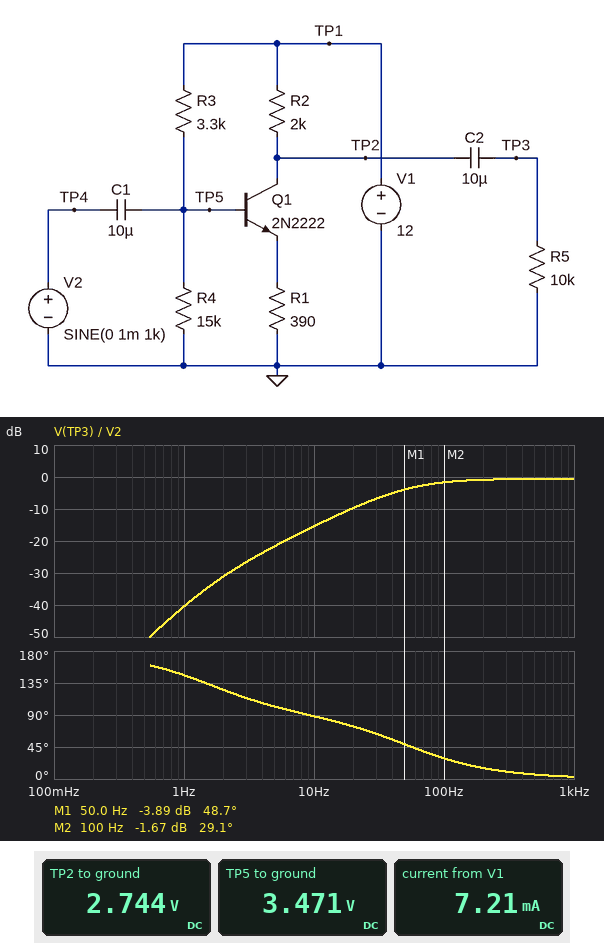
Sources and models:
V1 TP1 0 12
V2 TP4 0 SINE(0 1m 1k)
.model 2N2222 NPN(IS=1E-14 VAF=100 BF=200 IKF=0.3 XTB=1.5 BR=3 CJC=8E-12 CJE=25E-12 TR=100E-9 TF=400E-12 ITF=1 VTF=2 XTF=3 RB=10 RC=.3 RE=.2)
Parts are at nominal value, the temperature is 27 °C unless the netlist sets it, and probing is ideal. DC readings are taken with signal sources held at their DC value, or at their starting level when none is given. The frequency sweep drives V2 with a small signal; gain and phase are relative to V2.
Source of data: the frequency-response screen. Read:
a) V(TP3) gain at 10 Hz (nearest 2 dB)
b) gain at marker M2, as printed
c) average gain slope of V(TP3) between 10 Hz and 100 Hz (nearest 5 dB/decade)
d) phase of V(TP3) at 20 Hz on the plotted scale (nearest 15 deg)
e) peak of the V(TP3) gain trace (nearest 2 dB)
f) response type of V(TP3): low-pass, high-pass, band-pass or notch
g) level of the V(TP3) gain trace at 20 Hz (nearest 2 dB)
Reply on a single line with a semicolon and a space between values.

-16 dB; -1.67 dB; 15 dB/decade; 75 deg; 0 dB; high-pass; -10 dB
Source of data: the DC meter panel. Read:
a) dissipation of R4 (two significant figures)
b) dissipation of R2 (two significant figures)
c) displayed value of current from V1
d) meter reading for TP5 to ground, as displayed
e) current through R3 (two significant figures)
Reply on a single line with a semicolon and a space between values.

800 µW; 43 mW; 7.21 mA; 3.471 V; 2.6 mA
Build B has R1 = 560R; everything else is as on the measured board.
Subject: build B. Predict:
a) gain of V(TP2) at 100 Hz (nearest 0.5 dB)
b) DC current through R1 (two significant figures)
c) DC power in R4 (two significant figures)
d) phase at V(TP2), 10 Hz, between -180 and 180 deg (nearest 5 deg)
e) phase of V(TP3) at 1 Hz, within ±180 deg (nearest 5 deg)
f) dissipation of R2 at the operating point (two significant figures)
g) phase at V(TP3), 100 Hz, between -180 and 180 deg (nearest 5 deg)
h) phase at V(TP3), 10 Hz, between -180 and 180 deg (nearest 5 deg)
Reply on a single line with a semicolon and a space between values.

-1.0 dB; 6.3 mA; 1.2 mW; 75 deg; 145 deg; 36 mW; 25 deg; 85 deg
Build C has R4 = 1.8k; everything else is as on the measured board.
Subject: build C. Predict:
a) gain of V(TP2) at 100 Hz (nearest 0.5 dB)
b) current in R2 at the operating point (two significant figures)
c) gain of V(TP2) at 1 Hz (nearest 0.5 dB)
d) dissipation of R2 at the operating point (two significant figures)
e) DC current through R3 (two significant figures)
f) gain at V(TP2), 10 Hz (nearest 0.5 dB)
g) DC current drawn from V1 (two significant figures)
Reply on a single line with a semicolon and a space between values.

-2.5 dB; 4.8 mA; -36.5 dB; 47 mW; 2.7 mA; -16.5 dB; 7.6 mA
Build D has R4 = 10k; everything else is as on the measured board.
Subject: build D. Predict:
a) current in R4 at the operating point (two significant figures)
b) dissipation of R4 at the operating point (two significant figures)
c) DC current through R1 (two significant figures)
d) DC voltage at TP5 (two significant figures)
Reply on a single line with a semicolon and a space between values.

340 µA; 1.2 mW; 6.9 mA; 3.4 V
